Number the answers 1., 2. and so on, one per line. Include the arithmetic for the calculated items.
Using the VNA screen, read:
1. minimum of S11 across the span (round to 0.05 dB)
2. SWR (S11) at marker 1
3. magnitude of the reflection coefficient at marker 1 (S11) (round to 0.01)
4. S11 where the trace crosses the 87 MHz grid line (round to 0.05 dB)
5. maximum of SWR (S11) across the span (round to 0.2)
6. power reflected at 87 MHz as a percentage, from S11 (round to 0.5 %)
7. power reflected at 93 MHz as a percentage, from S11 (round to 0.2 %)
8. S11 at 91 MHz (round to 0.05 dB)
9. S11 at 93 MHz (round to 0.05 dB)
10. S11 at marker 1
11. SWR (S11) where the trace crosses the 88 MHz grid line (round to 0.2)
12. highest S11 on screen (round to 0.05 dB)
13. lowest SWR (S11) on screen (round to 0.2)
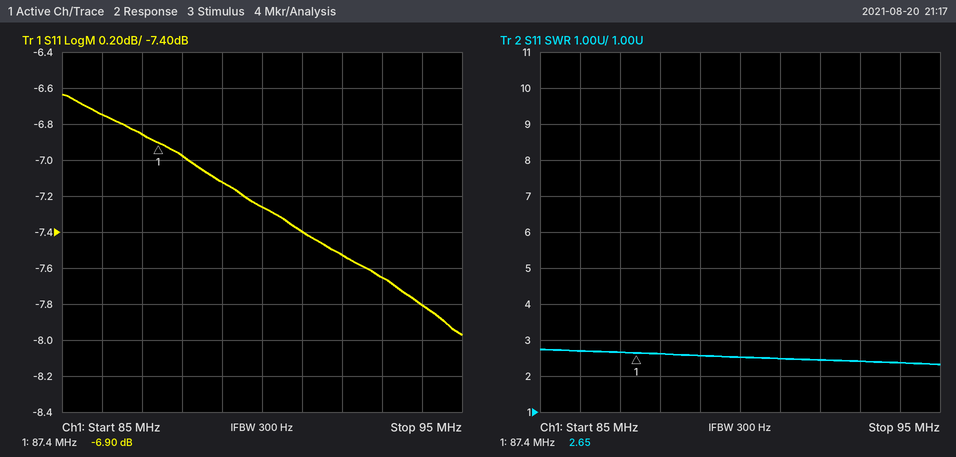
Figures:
1. -7.95 dB
2. 2.65
3. 10^(-6.9/20) ≈ 0.45
4. -6.85 dB
5. 2.8
6. 10^(-6.85/10) ≈ 20.7 %, so 20.5 % to the nearest 0.5 %
7. 10^(-7.65/10) ≈ 17.2 %
8. -7.40 dB
9. -7.65 dB
10. -6.90 dB
11. 2.6
12. -6.65 dB
13. 2.4
